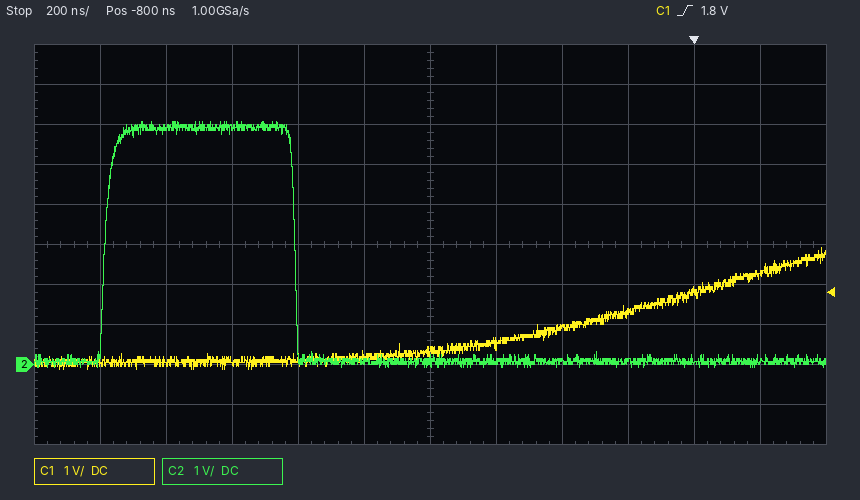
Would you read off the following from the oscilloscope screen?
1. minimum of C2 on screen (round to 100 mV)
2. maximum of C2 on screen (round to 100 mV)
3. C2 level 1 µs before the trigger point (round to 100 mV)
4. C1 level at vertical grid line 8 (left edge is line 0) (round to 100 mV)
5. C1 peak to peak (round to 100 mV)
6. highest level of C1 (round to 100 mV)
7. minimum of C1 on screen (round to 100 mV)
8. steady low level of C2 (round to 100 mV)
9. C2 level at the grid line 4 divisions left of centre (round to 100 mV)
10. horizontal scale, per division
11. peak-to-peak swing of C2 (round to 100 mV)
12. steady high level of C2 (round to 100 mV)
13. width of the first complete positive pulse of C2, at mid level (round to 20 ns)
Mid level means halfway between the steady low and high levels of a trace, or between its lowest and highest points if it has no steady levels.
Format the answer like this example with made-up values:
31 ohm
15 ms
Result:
-100 mV
6.1 V
100 mV
900 mV
3.0 V
2.9 V
-100 mV
100 mV
5.9 V
200 ns
6.2 V
5.9 V
580 ns
